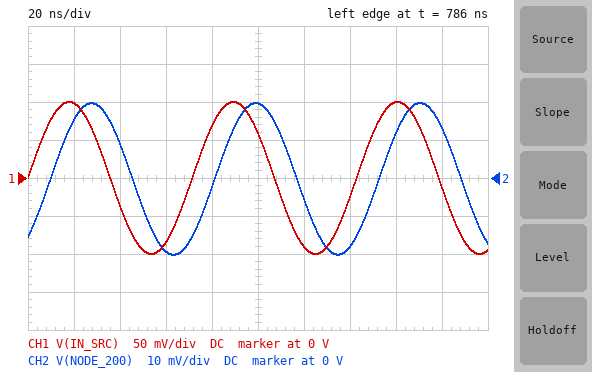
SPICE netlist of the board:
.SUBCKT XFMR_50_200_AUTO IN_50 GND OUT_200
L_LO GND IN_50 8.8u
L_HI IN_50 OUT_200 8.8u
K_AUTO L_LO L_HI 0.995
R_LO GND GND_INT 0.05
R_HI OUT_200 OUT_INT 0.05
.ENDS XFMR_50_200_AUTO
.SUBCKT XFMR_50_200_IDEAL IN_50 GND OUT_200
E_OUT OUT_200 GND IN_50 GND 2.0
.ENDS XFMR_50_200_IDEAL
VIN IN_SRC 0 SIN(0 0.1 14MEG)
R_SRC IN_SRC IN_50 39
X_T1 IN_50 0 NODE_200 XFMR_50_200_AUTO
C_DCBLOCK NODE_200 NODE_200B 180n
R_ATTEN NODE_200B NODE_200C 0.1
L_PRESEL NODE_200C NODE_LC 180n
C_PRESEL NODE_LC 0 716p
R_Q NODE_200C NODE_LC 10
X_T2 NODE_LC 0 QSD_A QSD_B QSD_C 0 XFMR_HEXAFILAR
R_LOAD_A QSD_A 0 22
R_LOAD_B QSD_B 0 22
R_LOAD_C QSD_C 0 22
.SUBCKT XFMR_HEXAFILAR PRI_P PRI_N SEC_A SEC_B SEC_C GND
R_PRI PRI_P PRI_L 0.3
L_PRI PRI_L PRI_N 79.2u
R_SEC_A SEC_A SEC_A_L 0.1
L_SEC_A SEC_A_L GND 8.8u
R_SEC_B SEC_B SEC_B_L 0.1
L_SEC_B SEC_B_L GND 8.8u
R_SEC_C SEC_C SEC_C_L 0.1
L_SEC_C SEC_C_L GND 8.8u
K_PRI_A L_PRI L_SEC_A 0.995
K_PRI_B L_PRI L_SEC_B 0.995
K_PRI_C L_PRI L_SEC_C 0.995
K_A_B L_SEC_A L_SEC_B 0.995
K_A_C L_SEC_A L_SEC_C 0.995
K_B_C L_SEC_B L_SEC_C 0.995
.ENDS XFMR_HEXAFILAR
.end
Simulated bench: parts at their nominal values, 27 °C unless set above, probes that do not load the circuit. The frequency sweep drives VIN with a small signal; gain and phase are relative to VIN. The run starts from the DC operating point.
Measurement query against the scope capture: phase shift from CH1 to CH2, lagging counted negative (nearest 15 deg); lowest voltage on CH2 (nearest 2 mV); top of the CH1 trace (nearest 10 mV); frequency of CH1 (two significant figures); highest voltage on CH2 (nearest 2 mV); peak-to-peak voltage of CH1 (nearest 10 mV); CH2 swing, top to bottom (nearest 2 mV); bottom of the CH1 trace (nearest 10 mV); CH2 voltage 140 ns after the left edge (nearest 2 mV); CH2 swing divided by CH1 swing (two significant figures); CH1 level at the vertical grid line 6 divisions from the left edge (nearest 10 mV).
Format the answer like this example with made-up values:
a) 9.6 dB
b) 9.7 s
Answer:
a) -45 deg
b) -20 mV
c) 100 mV
d) 14 MHz
e) 20 mV
f) 200 mV
g) 40 mV
h) -100 mV
i) -18 mV
j) 0.20
k) -90 mV
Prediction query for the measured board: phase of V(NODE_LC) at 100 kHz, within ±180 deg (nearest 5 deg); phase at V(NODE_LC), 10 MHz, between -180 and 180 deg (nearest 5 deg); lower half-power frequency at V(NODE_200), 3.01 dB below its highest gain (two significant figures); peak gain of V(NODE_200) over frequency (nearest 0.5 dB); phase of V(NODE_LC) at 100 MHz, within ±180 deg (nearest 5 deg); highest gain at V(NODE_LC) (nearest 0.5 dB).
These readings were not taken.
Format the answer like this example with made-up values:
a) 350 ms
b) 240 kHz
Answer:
a) 75 deg
b) -70 deg
c) 290 kHz
d) -4.5 dB
e) -110 deg
f) -4.5 dB
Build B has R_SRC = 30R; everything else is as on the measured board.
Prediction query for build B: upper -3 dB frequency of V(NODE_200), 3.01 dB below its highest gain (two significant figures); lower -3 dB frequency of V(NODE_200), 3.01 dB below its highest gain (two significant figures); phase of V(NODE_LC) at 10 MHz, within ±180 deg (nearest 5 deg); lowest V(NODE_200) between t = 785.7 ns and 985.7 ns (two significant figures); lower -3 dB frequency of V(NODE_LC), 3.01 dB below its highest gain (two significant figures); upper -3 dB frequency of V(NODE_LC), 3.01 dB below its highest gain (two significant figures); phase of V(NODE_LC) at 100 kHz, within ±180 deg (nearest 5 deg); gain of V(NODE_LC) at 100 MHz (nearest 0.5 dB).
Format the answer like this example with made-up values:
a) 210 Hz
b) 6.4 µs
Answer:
a) 5.9 MHz
b) 270 kHz
c) -65 deg
d) -26 mV
e) 260 kHz
f) 6.5 MHz
g) 75 deg
h) -30.0 dB
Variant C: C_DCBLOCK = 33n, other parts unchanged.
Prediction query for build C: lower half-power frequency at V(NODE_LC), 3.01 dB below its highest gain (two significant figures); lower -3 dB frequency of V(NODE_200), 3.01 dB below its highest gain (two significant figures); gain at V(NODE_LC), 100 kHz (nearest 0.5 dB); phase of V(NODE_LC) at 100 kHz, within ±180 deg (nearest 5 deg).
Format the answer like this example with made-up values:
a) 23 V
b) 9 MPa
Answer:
a) 230 kHz
b) 280 kHz
c) -8.0 dB
d) 125 deg
